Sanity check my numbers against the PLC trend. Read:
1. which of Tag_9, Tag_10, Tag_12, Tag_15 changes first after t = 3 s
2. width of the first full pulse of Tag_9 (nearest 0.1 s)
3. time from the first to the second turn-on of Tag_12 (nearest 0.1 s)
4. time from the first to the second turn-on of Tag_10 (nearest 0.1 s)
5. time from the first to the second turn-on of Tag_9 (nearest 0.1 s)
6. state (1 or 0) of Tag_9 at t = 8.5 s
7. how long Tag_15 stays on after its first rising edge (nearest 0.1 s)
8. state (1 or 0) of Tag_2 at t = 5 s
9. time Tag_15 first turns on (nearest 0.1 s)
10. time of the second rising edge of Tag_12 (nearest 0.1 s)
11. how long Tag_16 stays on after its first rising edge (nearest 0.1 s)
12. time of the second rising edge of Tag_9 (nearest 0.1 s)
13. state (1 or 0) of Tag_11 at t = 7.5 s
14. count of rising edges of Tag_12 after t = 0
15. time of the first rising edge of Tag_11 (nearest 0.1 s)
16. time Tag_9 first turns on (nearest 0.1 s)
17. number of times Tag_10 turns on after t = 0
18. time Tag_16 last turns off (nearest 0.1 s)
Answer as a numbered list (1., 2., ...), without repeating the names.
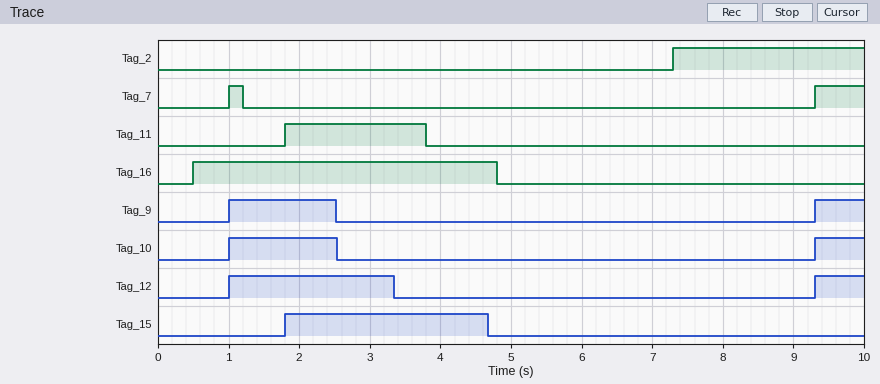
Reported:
1. Tag_12
2. 1.5 s
3. 8.3 s
4. 8.3 s
5. 8.3 s
6. 0
7. 2.9 s
8. 0
9. 1.8 s
10. 9.3 s
11. 4.3 s
12. 9.3 s
13. 0
14. 2
15. 1.8 s
16. 1.0 s
17. 2
18. 4.8 s
